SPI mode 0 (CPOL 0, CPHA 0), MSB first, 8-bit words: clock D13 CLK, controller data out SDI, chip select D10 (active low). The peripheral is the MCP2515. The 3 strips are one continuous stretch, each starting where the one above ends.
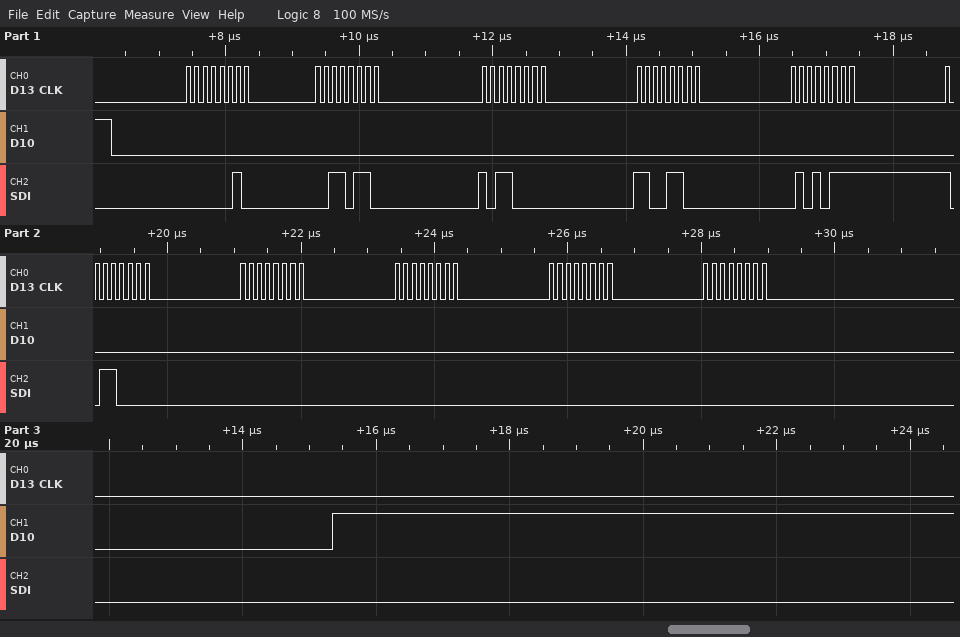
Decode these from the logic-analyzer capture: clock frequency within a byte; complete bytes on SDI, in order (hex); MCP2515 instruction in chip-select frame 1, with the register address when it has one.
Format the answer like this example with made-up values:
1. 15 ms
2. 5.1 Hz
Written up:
1. 8 MHz
2. 02 36 B0 CC 57 B0 00 00 00 00
3. WRITE 0x36
